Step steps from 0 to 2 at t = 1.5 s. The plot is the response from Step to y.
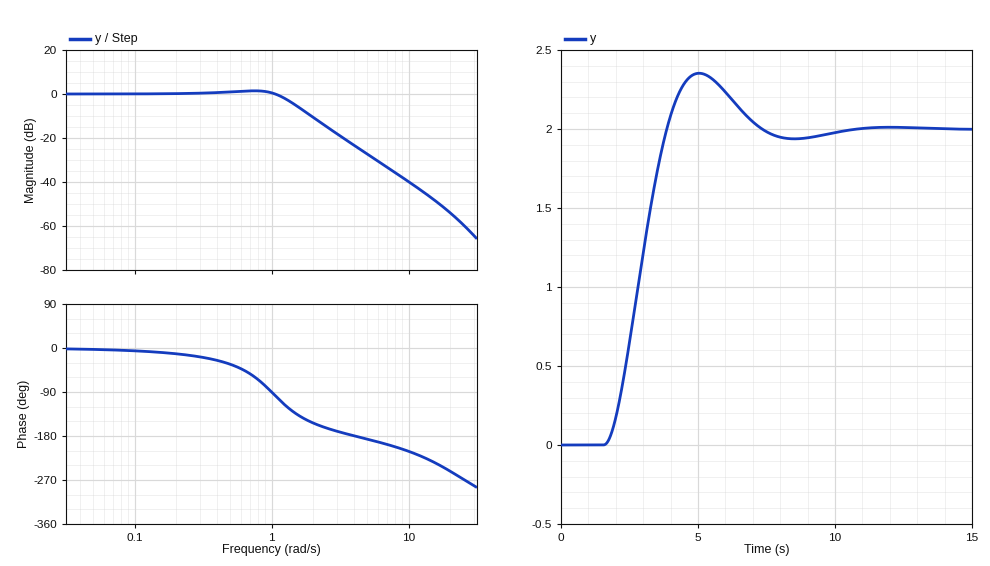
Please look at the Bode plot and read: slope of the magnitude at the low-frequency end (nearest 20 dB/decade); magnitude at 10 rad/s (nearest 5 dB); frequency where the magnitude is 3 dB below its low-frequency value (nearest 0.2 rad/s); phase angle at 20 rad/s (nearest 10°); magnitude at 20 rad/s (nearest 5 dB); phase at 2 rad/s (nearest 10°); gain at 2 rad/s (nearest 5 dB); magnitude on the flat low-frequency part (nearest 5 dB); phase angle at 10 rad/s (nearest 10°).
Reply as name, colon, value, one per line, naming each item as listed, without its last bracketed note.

slope of the magnitude at the low-frequency end: 0 dB/decade
magnitude at 10 rad/s: -40 dB
frequency where the magnitude is 3 dB below its low-frequency value: 1.4 rad/s
phase angle at 20 rad/s: -250°
magnitude at 20 rad/s: -55 dB
phase at 2 rad/s: -150°
gain at 2 rad/s: -10 dB
magnitude on the flat low-frequency part: 0 dB
phase angle at 10 rad/s: -210°
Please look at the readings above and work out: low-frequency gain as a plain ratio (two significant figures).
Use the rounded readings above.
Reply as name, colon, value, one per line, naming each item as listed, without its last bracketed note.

low-frequency gain as a plain ratio: 1.0
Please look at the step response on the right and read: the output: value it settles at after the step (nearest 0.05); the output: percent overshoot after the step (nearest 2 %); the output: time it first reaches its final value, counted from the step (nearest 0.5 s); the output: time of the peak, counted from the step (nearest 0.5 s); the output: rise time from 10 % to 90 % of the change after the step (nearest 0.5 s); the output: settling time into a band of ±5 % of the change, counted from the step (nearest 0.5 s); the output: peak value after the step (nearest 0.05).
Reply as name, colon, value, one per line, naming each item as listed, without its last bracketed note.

the output: value it settles at after the step: 2.00
the output: percent overshoot after the step: 18 %
the output: time it first reaches its final value, counted from the step: 2.5 s
the output: time of the peak, counted from the step: 3.5 s
the output: rise time from 10 % to 90 % of the change after the step: 1.5 s
the output: settling time into a band of ±5 % of the change, counted from the step: 5.0 s
the output: peak value after the step: 2.35
